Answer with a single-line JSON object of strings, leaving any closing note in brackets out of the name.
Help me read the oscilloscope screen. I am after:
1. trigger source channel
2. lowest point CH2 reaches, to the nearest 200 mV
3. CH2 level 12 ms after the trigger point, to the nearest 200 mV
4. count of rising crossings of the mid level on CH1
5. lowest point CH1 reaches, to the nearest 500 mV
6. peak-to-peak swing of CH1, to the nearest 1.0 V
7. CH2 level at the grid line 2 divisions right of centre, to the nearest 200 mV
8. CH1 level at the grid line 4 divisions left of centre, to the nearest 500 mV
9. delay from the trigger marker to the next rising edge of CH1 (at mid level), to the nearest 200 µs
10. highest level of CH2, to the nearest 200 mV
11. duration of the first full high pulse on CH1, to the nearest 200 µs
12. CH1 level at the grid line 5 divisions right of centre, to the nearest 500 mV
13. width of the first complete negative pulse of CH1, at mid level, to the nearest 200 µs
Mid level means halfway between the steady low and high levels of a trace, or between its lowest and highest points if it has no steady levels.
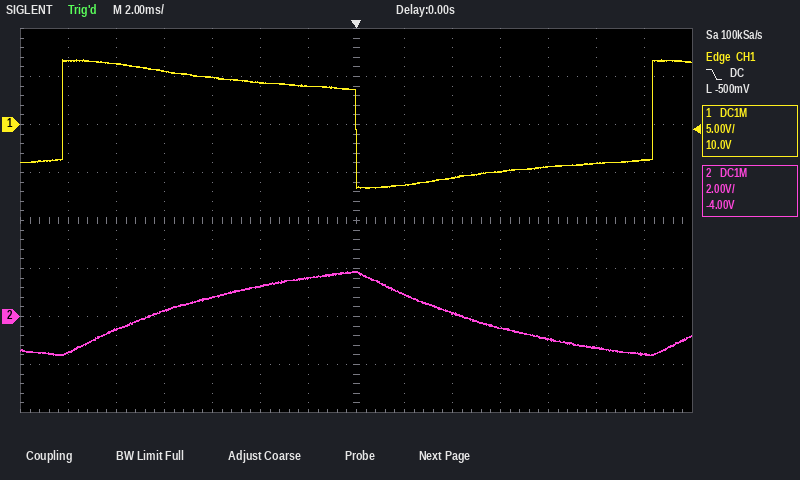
{"trigger source channel": "CH1", "lowest point CH2 reaches, to the nearest 200 mV": "-1.6 V", "CH2 level 12 ms after the trigger point, to the nearest 200 mV": "-1.6 V", "count of rising crossings of the mid level on CH1": "2", "lowest point CH1 reaches, to the nearest 500 mV": "-6.5 V", "peak-to-peak swing of CH1, to the nearest 1.0 V": "13.0 V", "CH2 level at the grid line 2 divisions right of centre, to the nearest 200 mV": "200 mV", "CH1 level at the grid line 4 divisions left of centre, to the nearest 500 mV": "5.5 V", "delay from the trigger marker to the next rising edge of CH1 (at mid level), to the nearest 200 µs": "12.4 ms", "highest level of CH2, to the nearest 200 mV": "1.8 V", "duration of the first full high pulse on CH1, to the nearest 200 µs": "12.2 ms", "CH1 level at the grid line 5 divisions right of centre, to the nearest 500 mV": "-4.0 V", "width of the first complete negative pulse of CH1, at mid level, to the nearest 200 µs": "12.4 ms"}
